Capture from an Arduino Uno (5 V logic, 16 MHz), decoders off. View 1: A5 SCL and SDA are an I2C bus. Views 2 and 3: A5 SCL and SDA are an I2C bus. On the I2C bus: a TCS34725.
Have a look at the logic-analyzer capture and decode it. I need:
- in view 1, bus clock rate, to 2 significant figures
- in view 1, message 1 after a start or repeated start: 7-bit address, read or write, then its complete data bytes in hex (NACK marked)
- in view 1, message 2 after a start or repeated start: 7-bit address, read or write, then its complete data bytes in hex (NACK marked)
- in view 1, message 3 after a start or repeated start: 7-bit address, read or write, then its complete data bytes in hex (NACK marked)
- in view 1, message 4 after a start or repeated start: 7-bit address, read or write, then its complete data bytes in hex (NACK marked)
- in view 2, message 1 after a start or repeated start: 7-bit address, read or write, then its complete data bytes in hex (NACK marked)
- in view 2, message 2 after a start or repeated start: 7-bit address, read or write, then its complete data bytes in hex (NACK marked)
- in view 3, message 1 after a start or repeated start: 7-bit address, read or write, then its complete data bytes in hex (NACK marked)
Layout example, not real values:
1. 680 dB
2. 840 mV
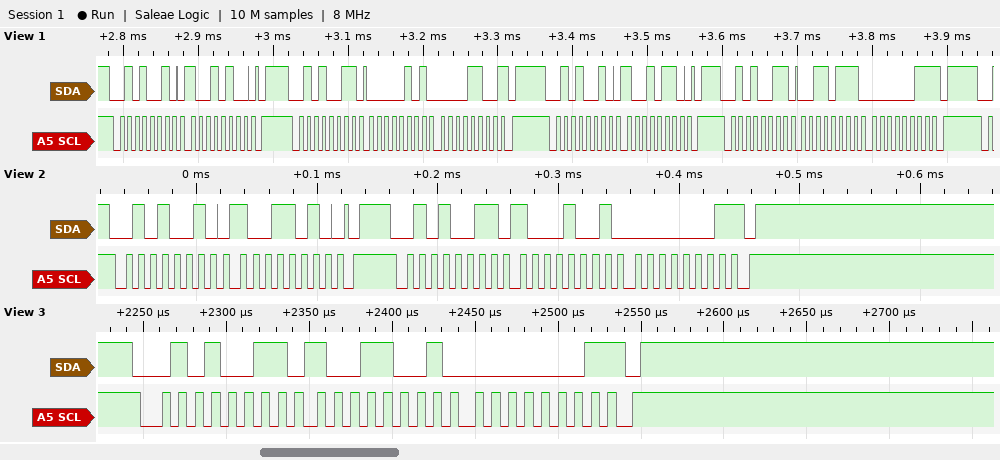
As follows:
1. 100 kHz
2. 0x29 write: 94
3. 0x29 read: 05 0C NACK
4. 0x29 write: 96
5. 0x29 read: 37 03 NACK
6. 0x29 write: 9A
7. 0x29 read: 89 01 NACK
8. 0x29 read: 99 01 NACK
